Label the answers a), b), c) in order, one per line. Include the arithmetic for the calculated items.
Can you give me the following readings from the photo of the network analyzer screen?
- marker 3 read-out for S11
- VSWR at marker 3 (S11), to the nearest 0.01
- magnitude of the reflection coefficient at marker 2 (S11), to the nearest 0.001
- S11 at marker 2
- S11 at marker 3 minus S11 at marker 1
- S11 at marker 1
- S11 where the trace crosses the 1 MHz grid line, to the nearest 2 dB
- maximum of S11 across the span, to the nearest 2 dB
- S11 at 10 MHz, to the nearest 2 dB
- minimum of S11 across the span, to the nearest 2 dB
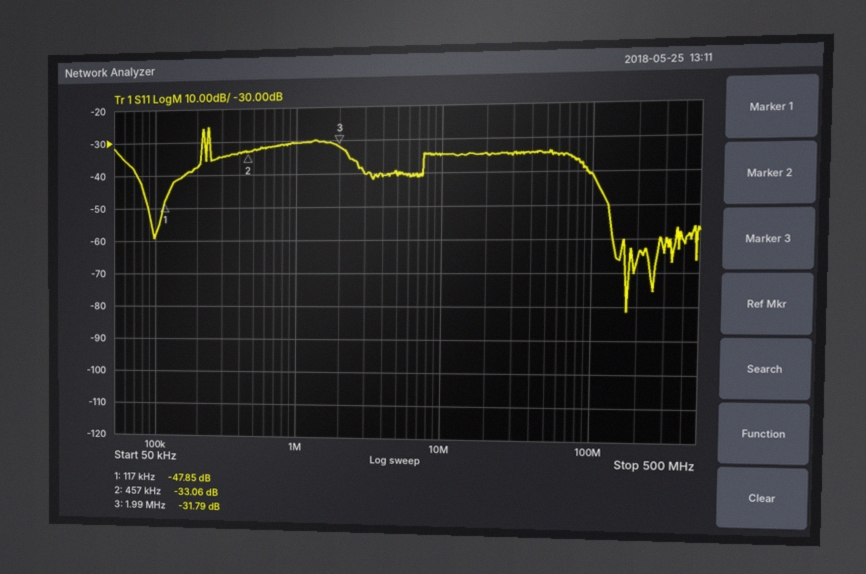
a) -31.79 dB
b) (1 + 0.0257)/(1 − 0.0257) ≈ 1.05
c) 10^(-33.06/20) ≈ 0.022
d) -33.06 dB
e) -31.79 − (-47.85) = 16.06 dB
f) -47.85 dB
g) -30 dB
h) -26 dB
i) -34 dB
j) -82 dB
